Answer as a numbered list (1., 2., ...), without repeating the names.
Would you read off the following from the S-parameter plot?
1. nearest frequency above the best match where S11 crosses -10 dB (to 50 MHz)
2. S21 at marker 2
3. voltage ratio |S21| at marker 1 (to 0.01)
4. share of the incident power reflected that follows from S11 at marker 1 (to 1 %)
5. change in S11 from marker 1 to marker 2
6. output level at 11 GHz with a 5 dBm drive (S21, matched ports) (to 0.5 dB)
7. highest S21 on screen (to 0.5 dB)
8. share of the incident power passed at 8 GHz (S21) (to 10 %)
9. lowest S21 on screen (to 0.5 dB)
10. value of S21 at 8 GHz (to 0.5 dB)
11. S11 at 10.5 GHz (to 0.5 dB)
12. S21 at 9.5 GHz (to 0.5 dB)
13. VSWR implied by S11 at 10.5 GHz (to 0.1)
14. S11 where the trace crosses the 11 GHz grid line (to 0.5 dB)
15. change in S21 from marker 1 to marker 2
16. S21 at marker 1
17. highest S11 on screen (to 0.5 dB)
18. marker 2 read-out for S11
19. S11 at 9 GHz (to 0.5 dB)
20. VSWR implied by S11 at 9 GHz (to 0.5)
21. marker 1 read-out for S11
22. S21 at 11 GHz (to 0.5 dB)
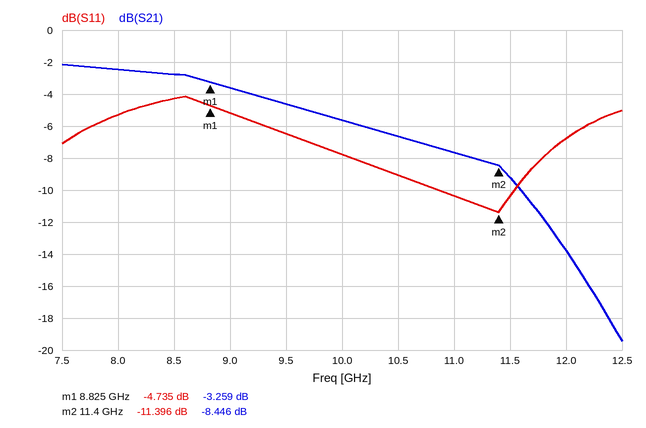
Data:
1. 11.55 GHz
2. -8.446 dB
3. 0.69
4. 34 %
5. -6.661 dB
6. -2.5 dBm
7. -2.0 dB
8. 60 %
9. -19.5 dB
10. -2.5 dB
11. -9.0 dB
12. -4.5 dB
13. 2.1
14. -10.5 dB
15. -5.187 dB
16. -3.259 dB
17. -4.0 dB
18. -11.396 dB
19. -5.0 dB
20. 3.5
21. -4.735 dB
22. -7.5 dB
